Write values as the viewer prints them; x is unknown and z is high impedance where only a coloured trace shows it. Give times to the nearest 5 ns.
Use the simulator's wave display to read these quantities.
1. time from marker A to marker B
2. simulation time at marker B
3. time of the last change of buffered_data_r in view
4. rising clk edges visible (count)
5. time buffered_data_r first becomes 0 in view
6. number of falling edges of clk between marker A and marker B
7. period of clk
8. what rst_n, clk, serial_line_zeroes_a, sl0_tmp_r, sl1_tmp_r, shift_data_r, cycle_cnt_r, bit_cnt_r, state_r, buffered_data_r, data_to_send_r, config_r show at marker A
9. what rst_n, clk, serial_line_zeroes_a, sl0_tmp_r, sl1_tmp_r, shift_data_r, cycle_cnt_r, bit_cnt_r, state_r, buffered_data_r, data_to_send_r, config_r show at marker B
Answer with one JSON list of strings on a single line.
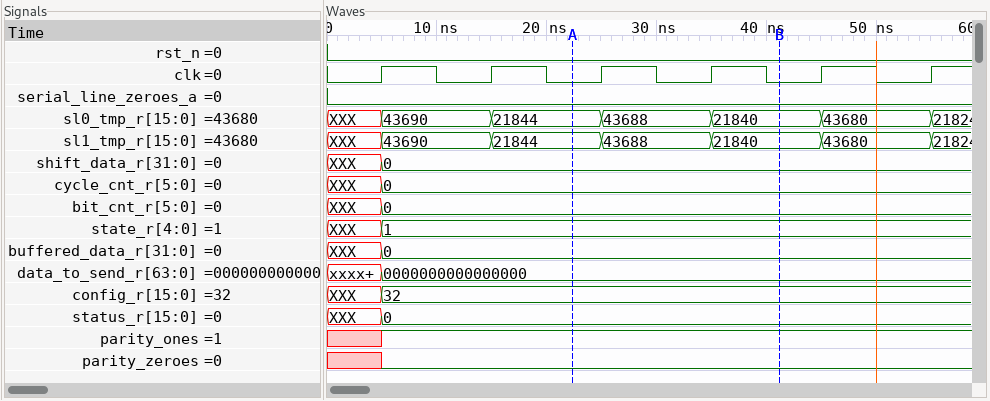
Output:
["20 ns", "40 ns", "5 ns", "6", "5 ns", "2", "10 ns", "rst_n=0, clk=0, serial_line_zeroes_a=0, sl0_tmp_r=21844, sl1_tmp_r=21844, shift_data_r=0, cycle_cnt_r=0, bit_cnt_r=0, state_r=1, buffered_data_r=0, data_to_send_r=0000000000000000, config_r=32", "rst_n=0, clk=0, serial_line_zeroes_a=0, sl0_tmp_r=21840, sl1_tmp_r=21840, shift_data_r=0, cycle_cnt_r=0, bit_cnt_r=0, state_r=1, buffered_data_r=0, data_to_send_r=0000000000000000, config_r=32"]
